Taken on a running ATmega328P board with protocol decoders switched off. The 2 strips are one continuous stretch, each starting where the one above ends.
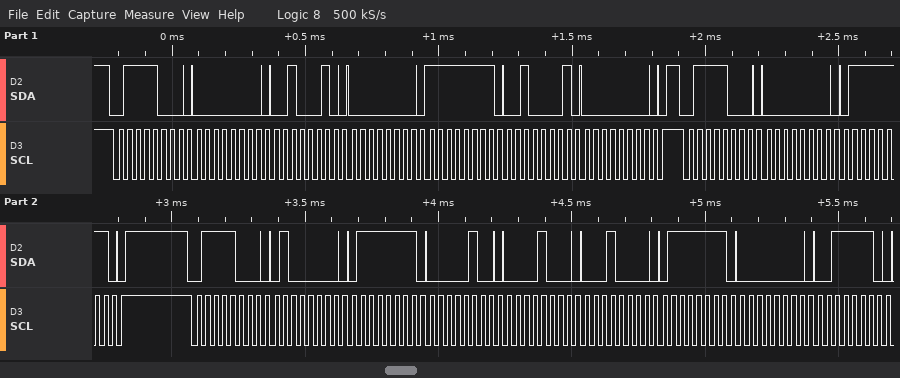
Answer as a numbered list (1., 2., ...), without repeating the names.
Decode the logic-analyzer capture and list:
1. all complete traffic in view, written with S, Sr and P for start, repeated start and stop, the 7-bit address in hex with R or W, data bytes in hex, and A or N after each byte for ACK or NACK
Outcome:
1. S 3CW A 00 A 22 A 00 A FF A 21 A 00 A P S 3CW A 00 A 7F A P S 3CW A 40 A 7F A 04 A 08 A 10 A 7F A 00 A 3E A
